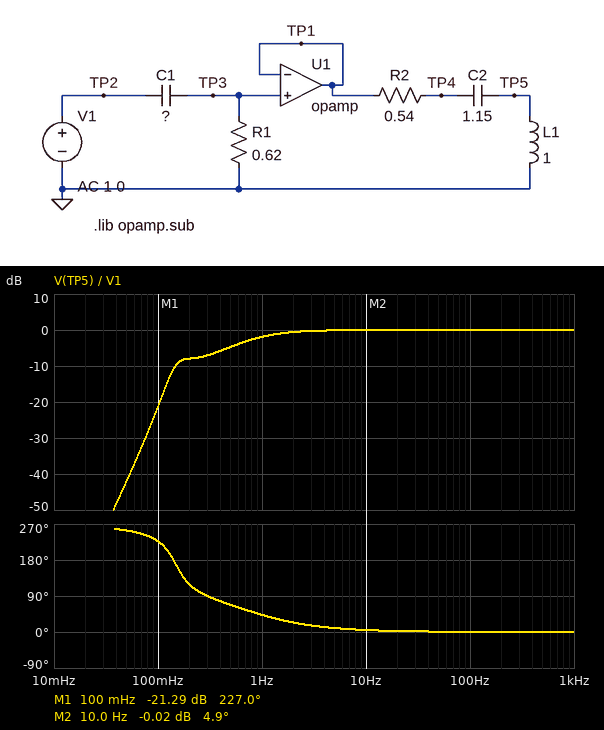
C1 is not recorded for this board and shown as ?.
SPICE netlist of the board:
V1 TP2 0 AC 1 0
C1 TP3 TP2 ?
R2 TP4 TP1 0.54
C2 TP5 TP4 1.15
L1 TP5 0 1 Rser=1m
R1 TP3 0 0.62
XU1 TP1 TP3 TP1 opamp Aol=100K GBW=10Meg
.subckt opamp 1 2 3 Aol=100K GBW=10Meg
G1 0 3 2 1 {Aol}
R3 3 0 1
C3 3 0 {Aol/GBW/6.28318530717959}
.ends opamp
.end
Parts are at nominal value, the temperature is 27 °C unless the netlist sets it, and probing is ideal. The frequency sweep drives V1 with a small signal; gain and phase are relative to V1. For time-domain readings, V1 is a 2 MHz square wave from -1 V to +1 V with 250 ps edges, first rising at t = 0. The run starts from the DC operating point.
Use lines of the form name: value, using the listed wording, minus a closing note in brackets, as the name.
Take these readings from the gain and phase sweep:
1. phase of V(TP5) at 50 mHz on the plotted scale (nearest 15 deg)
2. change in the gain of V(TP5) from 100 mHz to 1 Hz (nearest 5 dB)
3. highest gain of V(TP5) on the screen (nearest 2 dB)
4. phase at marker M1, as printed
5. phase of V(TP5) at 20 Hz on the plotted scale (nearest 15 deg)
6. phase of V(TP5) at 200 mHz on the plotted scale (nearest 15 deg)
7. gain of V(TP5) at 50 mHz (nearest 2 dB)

phase of V(TP5) at 50 mHz on the plotted scale: 255 deg
change in the gain of V(TP5) from 100 mHz to 1 Hz: 20 dB
highest gain of V(TP5) on the screen: 0 dB
phase at marker M1, as printed: 227.0 deg
phase of V(TP5) at 20 Hz on the plotted scale: 0 deg
phase of V(TP5) at 200 mHz on the plotted scale: 120 deg
gain of V(TP5) at 50 mHz: -42 dB
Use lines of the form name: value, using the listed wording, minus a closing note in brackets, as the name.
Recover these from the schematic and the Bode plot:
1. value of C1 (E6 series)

value of C1: 330 mF
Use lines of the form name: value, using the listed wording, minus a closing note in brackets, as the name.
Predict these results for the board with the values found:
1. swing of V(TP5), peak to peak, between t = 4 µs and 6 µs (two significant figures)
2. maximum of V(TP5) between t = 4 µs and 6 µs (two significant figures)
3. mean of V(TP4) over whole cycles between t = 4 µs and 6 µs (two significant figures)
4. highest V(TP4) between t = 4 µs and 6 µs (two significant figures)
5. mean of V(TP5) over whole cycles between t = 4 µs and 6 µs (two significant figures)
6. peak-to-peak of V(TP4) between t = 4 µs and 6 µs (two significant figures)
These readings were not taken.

swing of V(TP5), peak to peak, between t = 4 µs and 6 µs: 2.0 V
maximum of V(TP5) between t = 4 µs and 6 µs: 2.0 V
mean of V(TP4) over whole cycles between t = 4 µs and 6 µs: 1.0 V
highest V(TP4) between t = 4 µs and 6 µs: 2.0 V
mean of V(TP5) over whole cycles between t = 4 µs and 6 µs: 1.0 V
peak-to-peak of V(TP4) between t = 4 µs and 6 µs: 2.0 V
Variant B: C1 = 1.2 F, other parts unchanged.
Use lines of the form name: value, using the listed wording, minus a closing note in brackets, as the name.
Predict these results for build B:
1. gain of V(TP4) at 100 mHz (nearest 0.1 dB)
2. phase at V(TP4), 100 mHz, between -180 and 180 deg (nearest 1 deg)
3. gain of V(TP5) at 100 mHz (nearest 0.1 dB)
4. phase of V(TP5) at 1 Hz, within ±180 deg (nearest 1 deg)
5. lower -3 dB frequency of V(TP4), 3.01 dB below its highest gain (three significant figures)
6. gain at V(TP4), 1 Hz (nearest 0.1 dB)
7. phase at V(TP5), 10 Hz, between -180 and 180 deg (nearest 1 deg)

gain of V(TP4) at 100 mHz: -9.3 dB
phase at V(TP4), 100 mHz, between -180 and 180 deg: 29 deg
gain of V(TP5) at 100 mHz: -10.9 dB
phase of V(TP5) at 1 Hz, within ±180 deg: 17 deg
lower -3 dB frequency of V(TP4), 3.01 dB below its highest gain: 267 mHz
gain at V(TP4), 1 Hz: -0.2 dB
phase at V(TP5), 10 Hz, between -180 and 180 deg: 2 deg
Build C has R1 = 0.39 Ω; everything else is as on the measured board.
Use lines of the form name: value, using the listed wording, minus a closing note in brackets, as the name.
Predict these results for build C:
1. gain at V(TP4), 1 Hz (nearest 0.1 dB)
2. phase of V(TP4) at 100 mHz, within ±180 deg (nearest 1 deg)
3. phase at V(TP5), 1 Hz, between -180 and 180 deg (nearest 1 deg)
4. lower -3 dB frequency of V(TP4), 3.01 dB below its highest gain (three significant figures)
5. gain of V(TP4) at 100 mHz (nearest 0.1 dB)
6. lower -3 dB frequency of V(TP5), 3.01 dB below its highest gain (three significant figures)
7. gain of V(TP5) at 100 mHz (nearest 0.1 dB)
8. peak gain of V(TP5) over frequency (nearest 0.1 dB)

gain at V(TP4), 1 Hz: -4.1 dB
phase of V(TP4) at 100 mHz, within ±180 deg: 50 deg
phase at V(TP5), 1 Hz, between -180 and 180 deg: 56 deg
lower -3 dB frequency of V(TP4), 3.01 dB below its highest gain: 1.24 Hz
gain of V(TP4) at 100 mHz: -23.7 dB
lower -3 dB frequency of V(TP5), 3.01 dB below its highest gain: 1.21 Hz
gain of V(TP5) at 100 mHz: -25.3 dB
peak gain of V(TP5) over frequency: 0 dB
